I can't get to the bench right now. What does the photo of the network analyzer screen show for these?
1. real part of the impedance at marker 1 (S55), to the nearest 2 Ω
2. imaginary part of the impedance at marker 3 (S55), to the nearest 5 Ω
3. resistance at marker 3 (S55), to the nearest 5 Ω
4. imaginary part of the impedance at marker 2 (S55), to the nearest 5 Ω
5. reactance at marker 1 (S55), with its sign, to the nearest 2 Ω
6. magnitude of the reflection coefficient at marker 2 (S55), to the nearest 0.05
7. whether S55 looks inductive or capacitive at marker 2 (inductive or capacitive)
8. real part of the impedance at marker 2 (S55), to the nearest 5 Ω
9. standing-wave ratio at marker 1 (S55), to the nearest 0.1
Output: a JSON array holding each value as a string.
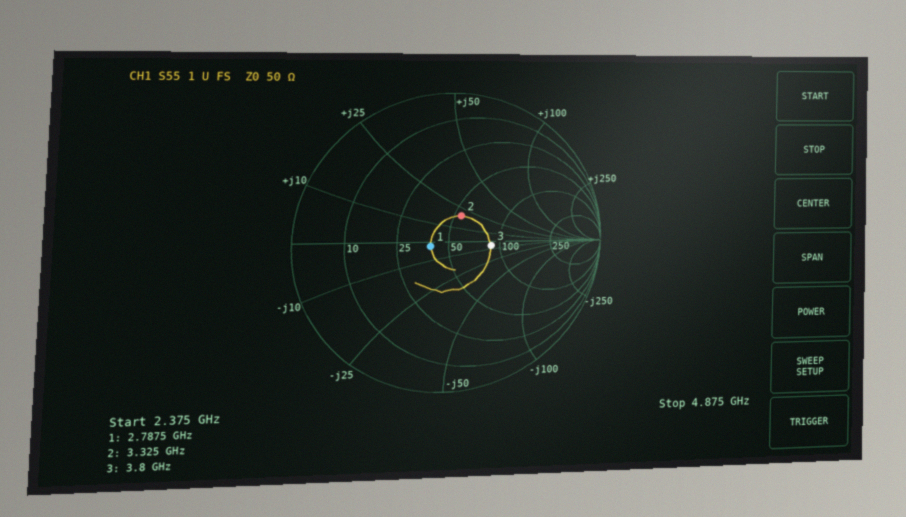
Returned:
["40 Ω", "-5 Ω", "90 Ω", "+20 Ω", "-2 Ω", "0.20", "inductive", "55 Ω", "1.3"]
